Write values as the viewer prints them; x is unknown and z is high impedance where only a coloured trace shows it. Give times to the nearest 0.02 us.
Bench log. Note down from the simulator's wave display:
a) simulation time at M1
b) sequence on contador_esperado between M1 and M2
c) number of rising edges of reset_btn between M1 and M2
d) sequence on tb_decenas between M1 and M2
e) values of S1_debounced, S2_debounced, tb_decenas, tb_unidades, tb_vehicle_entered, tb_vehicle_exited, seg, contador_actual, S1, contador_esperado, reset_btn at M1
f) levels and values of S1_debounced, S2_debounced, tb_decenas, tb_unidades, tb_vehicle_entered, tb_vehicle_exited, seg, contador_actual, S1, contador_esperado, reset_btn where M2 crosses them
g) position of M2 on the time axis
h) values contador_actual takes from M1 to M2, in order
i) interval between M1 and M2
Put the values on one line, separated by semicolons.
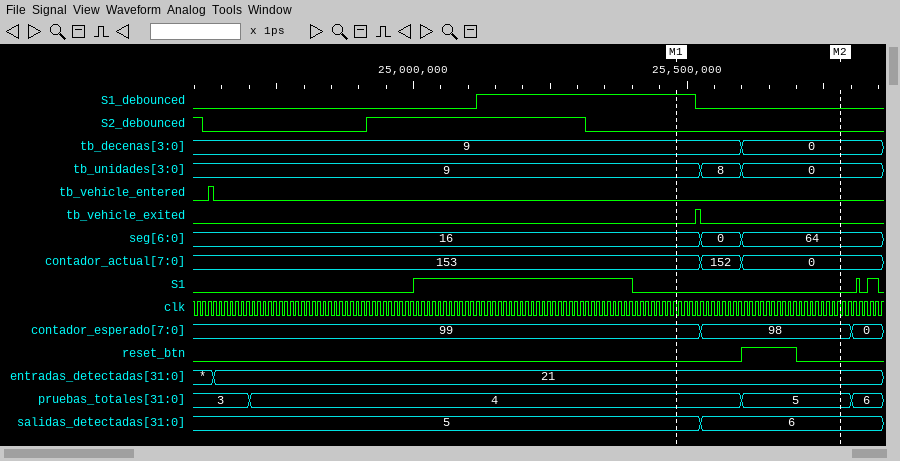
25.48 us; 99, 98; 1; 9, 0; S1_debounced=1, S2_debounced=0, tb_decenas=9, tb_unidades=9, tb_vehicle_entered=0, tb_vehicle_exited=0, seg=16, contador_actual=153, S1=0, contador_esperado=99, reset_btn=0; S1_debounced=0, S2_debounced=0, tb_decenas=0, tb_unidades=0, tb_vehicle_entered=0, tb_vehicle_exited=0, seg=64, contador_actual=0, S1=0, contador_esperado=98, reset_btn=0; 25.78 us; 153, 152, 0; 0.3 us
